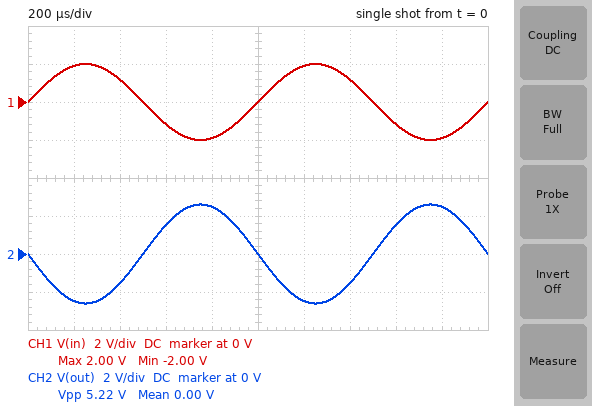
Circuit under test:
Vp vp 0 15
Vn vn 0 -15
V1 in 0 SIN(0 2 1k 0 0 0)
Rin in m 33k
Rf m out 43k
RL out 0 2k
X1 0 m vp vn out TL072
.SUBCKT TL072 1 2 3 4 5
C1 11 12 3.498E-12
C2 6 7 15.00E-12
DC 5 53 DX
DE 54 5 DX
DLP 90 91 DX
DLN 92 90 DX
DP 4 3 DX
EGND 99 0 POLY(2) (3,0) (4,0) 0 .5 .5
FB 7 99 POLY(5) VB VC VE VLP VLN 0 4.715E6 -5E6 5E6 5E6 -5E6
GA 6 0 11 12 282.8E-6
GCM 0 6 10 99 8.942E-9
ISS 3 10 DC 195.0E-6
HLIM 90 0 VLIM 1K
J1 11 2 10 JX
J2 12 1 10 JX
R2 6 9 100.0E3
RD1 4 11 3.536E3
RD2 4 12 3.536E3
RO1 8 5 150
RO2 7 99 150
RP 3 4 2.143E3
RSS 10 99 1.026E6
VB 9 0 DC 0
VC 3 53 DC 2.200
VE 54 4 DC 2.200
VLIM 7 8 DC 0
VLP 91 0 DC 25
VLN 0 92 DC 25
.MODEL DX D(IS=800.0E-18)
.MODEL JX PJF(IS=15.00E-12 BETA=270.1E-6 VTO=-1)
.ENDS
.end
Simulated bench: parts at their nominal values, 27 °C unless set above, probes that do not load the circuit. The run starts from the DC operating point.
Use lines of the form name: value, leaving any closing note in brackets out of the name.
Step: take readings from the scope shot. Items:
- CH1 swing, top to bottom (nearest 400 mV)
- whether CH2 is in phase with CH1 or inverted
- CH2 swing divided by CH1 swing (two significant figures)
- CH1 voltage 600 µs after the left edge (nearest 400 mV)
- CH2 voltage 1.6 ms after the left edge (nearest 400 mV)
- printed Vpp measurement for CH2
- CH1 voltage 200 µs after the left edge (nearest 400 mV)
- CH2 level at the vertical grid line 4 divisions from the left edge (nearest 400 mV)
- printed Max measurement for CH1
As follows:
CH1 swing, top to bottom: 4.0 V
whether CH2 is in phase with CH1 or inverted: inverted
CH2 swing divided by CH1 swing: 1.3
CH1 voltage 600 µs after the left edge: -1.2 V
CH2 voltage 1.6 ms after the left edge: 1.6 V
printed Vpp measurement for CH2: 5.22 V
CH1 voltage 200 µs after the left edge: 2.0 V
CH2 level at the vertical grid line 4 divisions from the left edge: 2.4 V
printed Max measurement for CH1: 2.00 V
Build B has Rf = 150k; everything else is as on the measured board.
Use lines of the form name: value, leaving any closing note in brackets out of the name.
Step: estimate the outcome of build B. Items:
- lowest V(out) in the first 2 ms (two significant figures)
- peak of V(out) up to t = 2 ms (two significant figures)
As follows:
lowest V(out) in the first 2 ms: -9.1 V
peak of V(out) up to t = 2 ms: 9.1 V
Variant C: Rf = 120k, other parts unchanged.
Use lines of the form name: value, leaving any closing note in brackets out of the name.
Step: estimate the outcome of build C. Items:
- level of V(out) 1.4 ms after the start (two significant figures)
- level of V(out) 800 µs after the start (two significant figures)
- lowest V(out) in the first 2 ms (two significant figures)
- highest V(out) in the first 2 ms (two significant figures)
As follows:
level of V(out) 1.4 ms after the start: -4.3 V
level of V(out) 800 µs after the start: 6.9 V
lowest V(out) in the first 2 ms: -7.3 V
highest V(out) in the first 2 ms: 7.3 V
